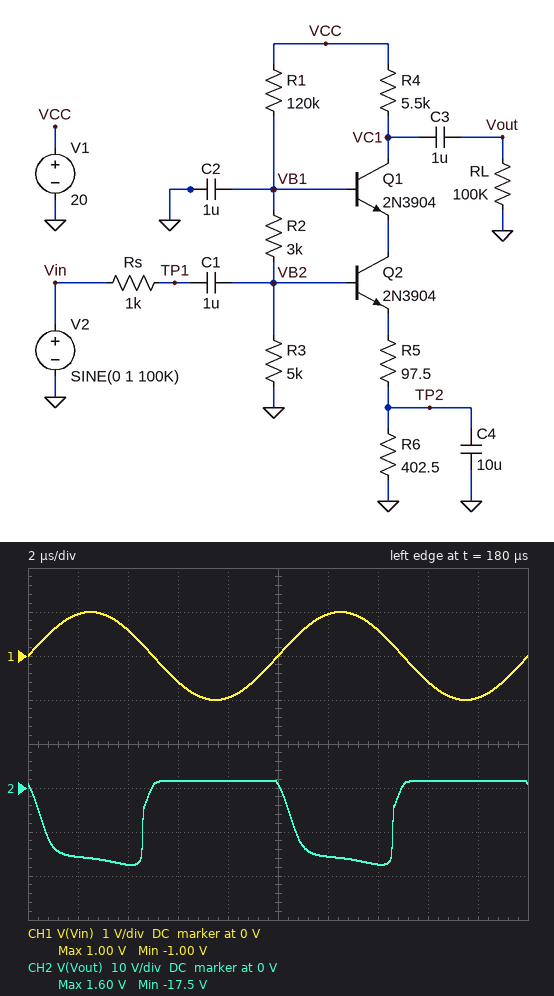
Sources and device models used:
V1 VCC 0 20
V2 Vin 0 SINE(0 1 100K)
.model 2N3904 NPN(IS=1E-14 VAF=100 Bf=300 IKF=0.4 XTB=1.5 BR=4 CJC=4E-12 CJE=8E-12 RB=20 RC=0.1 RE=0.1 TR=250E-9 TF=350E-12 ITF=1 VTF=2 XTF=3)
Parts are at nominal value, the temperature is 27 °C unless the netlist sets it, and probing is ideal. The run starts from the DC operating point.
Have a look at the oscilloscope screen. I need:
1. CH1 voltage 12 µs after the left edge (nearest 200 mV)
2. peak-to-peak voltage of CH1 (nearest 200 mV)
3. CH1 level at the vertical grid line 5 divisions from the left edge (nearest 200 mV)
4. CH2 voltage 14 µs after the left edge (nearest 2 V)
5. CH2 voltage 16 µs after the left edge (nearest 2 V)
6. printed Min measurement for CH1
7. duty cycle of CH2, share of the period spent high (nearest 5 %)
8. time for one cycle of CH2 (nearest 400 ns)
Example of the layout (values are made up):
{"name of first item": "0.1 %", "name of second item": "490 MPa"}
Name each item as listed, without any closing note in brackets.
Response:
{"CH1 voltage 12 µs after the left edge": "1.0 V", "peak-to-peak voltage of CH1": "2.0 V", "CH1 level at the vertical grid line 5 divisions from the left edge": "0 V", "CH2 voltage 14 µs after the left edge": "-18 V", "CH2 voltage 16 µs after the left edge": "2 V", "printed Min measurement for CH1": "-1.00 V", "duty cycle of CH2, share of the period spent high": "60 %", "time for one cycle of CH2": "10.0 µs"}
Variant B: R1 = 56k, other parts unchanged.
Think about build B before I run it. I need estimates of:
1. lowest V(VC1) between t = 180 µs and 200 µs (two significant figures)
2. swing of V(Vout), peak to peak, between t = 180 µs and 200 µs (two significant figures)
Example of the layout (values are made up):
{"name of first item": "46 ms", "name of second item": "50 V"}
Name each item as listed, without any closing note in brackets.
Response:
{"lowest V(VC1) between t = 180 µs and 200 µs": "1.5 V", "swing of V(Vout), peak to peak, between t = 180 µs and 200 µs": "18 V"}
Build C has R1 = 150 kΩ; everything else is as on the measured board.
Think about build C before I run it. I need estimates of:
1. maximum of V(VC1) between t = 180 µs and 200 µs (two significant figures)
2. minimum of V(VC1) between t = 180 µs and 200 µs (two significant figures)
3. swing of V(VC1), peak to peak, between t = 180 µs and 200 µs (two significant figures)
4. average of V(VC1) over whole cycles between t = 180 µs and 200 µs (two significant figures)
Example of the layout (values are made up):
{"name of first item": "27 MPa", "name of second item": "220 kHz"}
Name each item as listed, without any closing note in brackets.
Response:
{"maximum of V(VC1) between t = 180 µs and 200 µs": "20 V", "minimum of V(VC1) between t = 180 µs and 200 µs": "6.8 V", "swing of V(VC1), peak to peak, between t = 180 µs and 200 µs": "13 V", "average of V(VC1) over whole cycles between t = 180 µs and 200 µs": "15 V"}
